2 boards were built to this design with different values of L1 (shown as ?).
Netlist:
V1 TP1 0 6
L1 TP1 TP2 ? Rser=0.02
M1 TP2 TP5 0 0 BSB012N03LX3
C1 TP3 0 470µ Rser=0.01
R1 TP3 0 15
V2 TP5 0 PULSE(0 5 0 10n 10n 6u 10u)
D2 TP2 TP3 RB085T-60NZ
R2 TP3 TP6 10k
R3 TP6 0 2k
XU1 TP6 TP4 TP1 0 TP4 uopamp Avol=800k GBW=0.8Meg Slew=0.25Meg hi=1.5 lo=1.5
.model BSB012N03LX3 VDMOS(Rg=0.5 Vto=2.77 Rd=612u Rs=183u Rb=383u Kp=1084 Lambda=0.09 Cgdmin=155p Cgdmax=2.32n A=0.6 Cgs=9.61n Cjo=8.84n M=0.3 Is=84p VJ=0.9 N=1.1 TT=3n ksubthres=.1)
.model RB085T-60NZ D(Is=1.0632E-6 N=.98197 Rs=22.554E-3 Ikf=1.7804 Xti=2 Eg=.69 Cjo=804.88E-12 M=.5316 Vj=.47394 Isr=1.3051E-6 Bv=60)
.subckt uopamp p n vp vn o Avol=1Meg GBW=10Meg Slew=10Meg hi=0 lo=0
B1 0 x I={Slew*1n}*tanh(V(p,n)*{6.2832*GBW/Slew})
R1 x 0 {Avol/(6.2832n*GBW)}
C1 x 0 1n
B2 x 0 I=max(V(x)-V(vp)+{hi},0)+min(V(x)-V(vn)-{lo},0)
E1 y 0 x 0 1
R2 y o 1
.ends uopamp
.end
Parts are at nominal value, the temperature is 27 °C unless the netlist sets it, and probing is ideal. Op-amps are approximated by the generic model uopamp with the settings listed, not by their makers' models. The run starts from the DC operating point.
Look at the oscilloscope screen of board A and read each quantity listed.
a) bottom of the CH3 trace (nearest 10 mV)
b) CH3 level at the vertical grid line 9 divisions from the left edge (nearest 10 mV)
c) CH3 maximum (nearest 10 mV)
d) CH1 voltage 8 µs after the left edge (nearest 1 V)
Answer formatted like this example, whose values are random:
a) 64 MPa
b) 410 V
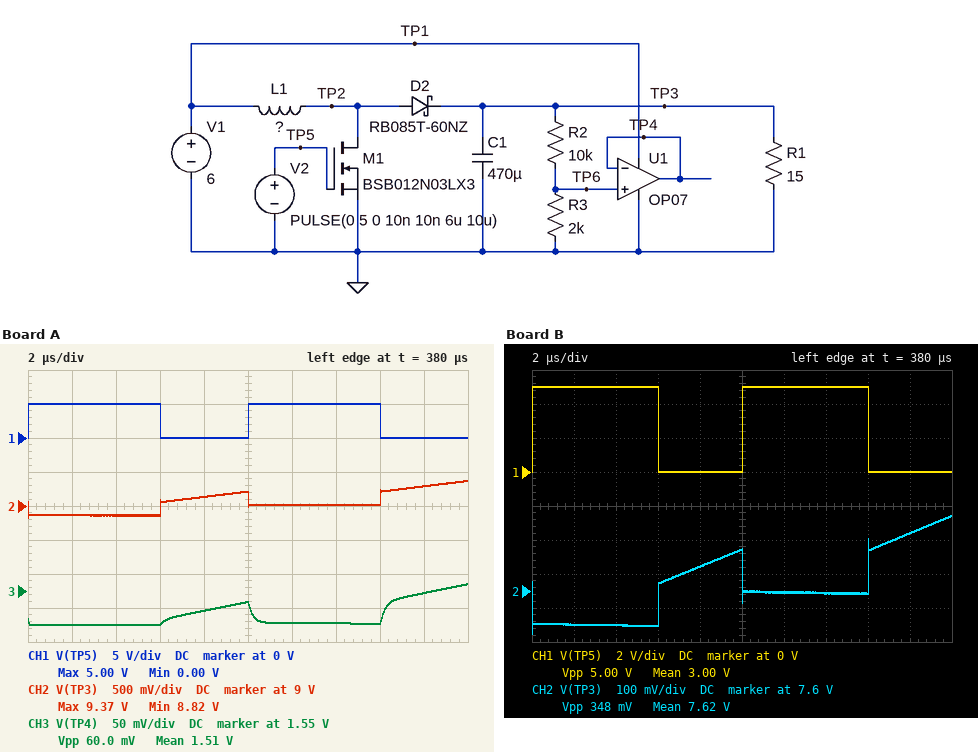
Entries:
a) 1.50 V
b) 1.55 V
c) 1.56 V
d) 0 V
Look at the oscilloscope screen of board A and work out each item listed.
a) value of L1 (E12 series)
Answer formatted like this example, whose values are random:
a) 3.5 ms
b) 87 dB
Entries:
a) 56 µH
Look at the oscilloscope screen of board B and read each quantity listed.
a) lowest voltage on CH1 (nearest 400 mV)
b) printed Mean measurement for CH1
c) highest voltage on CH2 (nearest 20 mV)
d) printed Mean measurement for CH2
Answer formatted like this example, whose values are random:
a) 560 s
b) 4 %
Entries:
a) 0 V
b) 3.00 V
c) 7.82 V
d) 7.62 V
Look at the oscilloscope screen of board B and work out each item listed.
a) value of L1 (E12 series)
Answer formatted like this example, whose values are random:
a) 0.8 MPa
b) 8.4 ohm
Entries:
a) 100 µH
